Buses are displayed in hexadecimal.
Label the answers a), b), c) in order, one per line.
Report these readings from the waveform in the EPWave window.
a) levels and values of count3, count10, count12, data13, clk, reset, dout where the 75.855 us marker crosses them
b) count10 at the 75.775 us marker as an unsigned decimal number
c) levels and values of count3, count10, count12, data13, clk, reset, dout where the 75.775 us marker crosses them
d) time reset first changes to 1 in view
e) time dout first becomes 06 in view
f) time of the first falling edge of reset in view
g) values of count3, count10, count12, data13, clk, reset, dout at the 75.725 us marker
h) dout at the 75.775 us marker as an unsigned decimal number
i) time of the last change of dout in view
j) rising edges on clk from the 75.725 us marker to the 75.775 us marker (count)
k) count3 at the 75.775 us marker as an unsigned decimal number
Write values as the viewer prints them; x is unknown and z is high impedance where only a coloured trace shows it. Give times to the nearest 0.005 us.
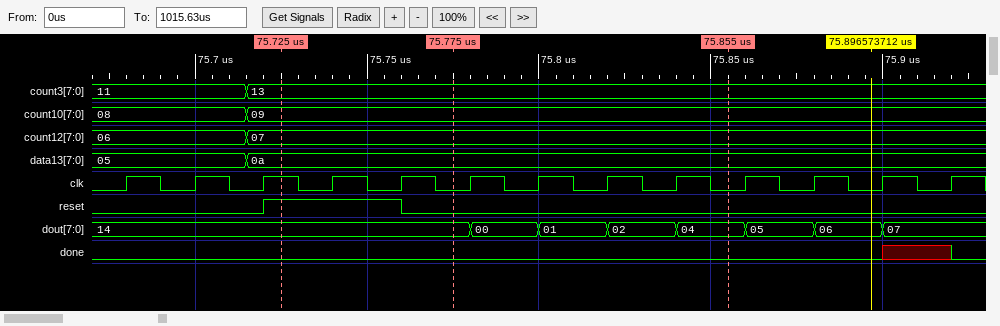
a) count3=13, count10=09, count12=07, data13=0a, clk=0, reset=0, dout=04
b) 9
c) count3=13, count10=09, count12=07, data13=0a, clk=0, reset=0, dout=14
d) 75.72 us
e) 75.88 us
f) 75.76 us
g) count3=13, count10=09, count12=07, data13=0a, clk=1, reset=1, dout=14
h) 20
i) 75.9 us
j) 2
k) 19
